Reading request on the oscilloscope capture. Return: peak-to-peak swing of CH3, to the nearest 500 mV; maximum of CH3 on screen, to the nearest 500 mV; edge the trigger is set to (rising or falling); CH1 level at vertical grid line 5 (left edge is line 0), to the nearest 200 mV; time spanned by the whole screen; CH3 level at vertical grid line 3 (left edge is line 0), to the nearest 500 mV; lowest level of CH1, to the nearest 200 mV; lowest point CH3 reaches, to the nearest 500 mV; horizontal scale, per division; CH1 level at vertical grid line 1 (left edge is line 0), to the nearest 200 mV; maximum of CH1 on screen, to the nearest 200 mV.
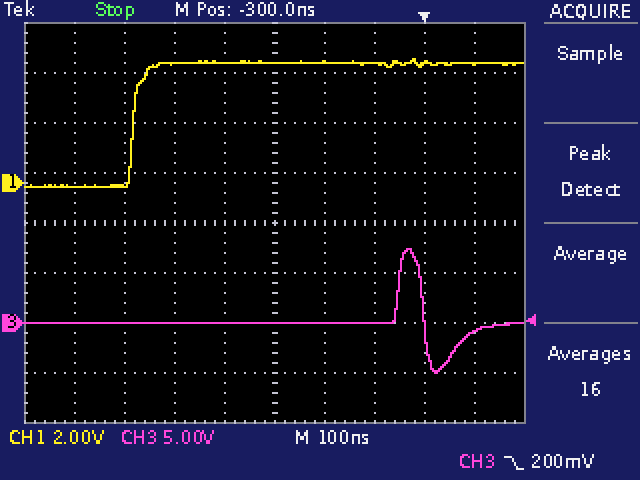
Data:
12.5 V
7.5 V
falling
4.8 V
1 µs
0.0 V
-200 mV
-5.0 V
100 ns
-200 mV
5.0 V
